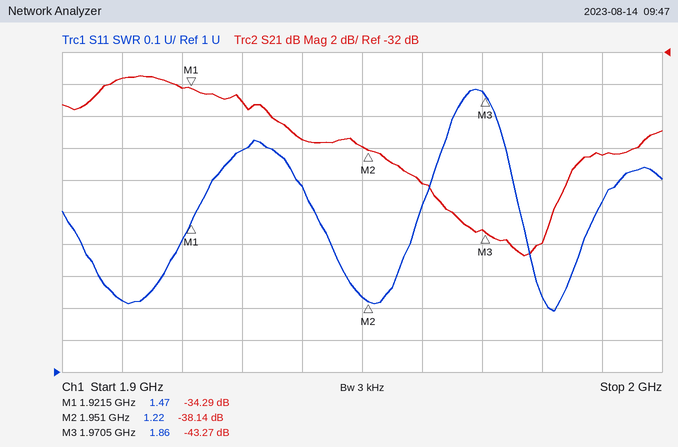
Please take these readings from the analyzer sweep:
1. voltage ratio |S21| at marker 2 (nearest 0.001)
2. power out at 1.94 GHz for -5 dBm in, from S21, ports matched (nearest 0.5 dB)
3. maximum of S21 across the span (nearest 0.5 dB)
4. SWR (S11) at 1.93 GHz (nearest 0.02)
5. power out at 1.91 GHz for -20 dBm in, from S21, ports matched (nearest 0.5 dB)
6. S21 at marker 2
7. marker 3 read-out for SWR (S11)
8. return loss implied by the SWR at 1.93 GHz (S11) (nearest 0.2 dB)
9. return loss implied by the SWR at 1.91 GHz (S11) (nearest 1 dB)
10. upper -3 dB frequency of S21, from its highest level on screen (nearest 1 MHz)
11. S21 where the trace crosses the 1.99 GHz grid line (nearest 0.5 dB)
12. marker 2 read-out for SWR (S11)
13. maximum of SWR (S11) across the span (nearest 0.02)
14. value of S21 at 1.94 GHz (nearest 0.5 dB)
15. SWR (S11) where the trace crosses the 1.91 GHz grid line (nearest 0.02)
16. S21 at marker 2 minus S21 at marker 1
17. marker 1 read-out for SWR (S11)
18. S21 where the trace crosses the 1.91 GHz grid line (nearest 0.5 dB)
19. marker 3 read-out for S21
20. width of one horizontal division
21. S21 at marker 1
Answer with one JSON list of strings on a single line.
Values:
["0.012", "-42.5 dBm", "-33.5 dB", "1.70", "-53.5 dBm", "-38.14 dB", "1.86", "11.8 dB", "20 dB", "1.937 GHz", "-38.5 dB", "1.22", "1.88", "-37.5 dB", "1.22", "-3.85 dB", "1.47", "-33.5 dB", "-43.27 dB", "10 MHz", "-34.29 dB"]
